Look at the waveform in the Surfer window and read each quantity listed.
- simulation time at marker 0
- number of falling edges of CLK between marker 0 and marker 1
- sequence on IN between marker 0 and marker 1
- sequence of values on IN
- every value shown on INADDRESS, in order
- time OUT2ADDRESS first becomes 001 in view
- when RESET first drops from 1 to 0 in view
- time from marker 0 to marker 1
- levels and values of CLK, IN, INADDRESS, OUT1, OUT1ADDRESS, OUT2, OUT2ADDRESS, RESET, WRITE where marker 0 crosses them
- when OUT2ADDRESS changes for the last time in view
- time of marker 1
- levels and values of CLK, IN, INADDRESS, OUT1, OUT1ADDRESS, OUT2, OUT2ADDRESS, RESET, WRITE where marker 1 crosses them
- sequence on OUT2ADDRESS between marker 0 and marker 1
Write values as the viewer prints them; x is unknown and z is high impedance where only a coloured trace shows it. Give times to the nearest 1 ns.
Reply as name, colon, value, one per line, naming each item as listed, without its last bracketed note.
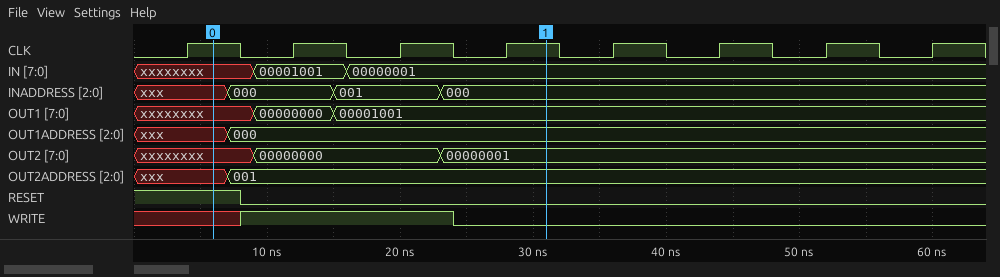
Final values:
simulation time at marker 0: 6 ns
number of falling edges of CLK between marker 0 and marker 1: 3
sequence on IN between marker 0 and marker 1: xxxxxxxx, 00001001, 00000001
sequence of values on IN: xxxxxxxx, 00001001, 00000001
every value shown on INADDRESS, in order: xxx, 000, 001, 000
time OUT2ADDRESS first becomes 001 in view: 7 ns
when RESET first drops from 1 to 0 in view: 8 ns
time from marker 0 to marker 1: 25 ns
levels and values of CLK, IN, INADDRESS, OUT1, OUT1ADDRESS, OUT2, OUT2ADDRESS, RESET, WRITE where marker 0 crosses them: CLK=1, IN=xxxxxxxx, INADDRESS=xxx, OUT1=xxxxxxxx, OUT1ADDRESS=xxx, OUT2=xxxxxxxx, OUT2ADDRESS=xxx, RESET=1, WRITE=x
when OUT2ADDRESS changes for the last time in view: 7 ns
time of marker 1: 31 ns
levels and values of CLK, IN, INADDRESS, OUT1, OUT1ADDRESS, OUT2, OUT2ADDRESS, RESET, WRITE where marker 1 crosses them: CLK=1, IN=00000001, INADDRESS=000, OUT1=00001001, OUT1ADDRESS=000, OUT2=00000001, OUT2ADDRESS=001, RESET=0, WRITE=0
sequence on OUT2ADDRESS between marker 0 and marker 1: xxx, 001
